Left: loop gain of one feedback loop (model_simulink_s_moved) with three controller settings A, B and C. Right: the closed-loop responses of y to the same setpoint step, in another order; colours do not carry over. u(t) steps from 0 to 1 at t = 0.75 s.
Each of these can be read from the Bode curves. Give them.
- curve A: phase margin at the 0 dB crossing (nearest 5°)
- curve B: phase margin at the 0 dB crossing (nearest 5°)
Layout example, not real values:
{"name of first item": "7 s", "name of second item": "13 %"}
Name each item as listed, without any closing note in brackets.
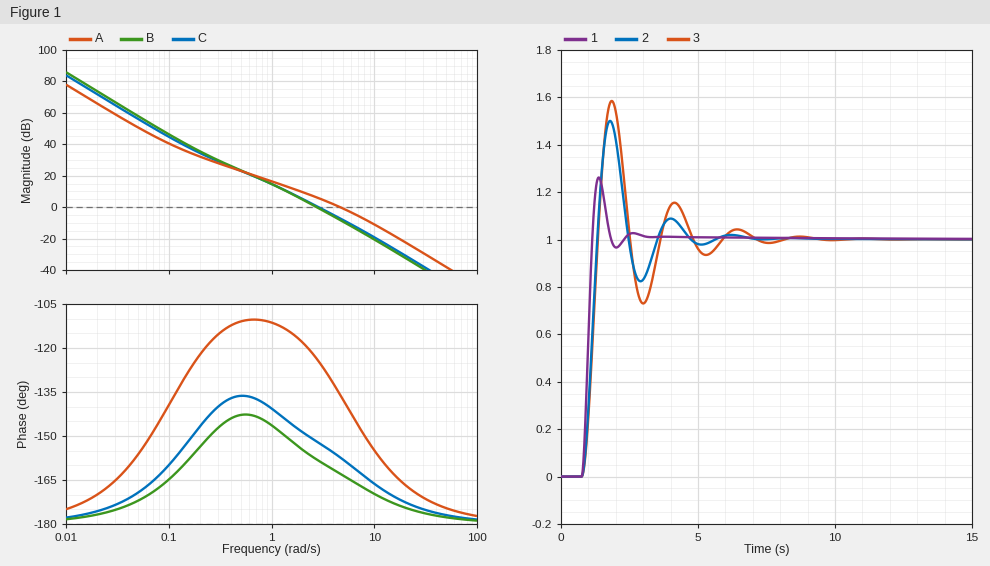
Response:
{"curve A: phase margin at the 0 dB crossing": "45°", "curve B: phase margin at the 0 dB crossing": "20°"}
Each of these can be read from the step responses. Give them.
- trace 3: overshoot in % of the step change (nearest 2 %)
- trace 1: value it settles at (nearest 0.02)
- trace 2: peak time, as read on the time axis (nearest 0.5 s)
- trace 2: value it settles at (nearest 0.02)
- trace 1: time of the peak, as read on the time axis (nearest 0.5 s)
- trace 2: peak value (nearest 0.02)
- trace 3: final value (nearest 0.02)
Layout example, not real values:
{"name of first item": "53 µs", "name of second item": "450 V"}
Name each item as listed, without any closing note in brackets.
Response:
{"trace 3: overshoot in % of the step change": "58 %", "trace 1: value it settles at": "1.00", "trace 2: peak time, as read on the time axis": "2.0 s", "trace 2: value it settles at": "1.00", "trace 1: time of the peak, as read on the time axis": "1.5 s", "trace 2: peak value": "1.50", "trace 3: final value": "1.00"}
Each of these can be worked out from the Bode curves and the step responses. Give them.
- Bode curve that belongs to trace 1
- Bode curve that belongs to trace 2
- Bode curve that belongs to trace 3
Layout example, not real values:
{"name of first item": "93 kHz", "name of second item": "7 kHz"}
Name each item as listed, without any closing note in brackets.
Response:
{"Bode curve that belongs to trace 1": "A", "Bode curve that belongs to trace 2": "C", "Bode curve that belongs to trace 3": "B"}
